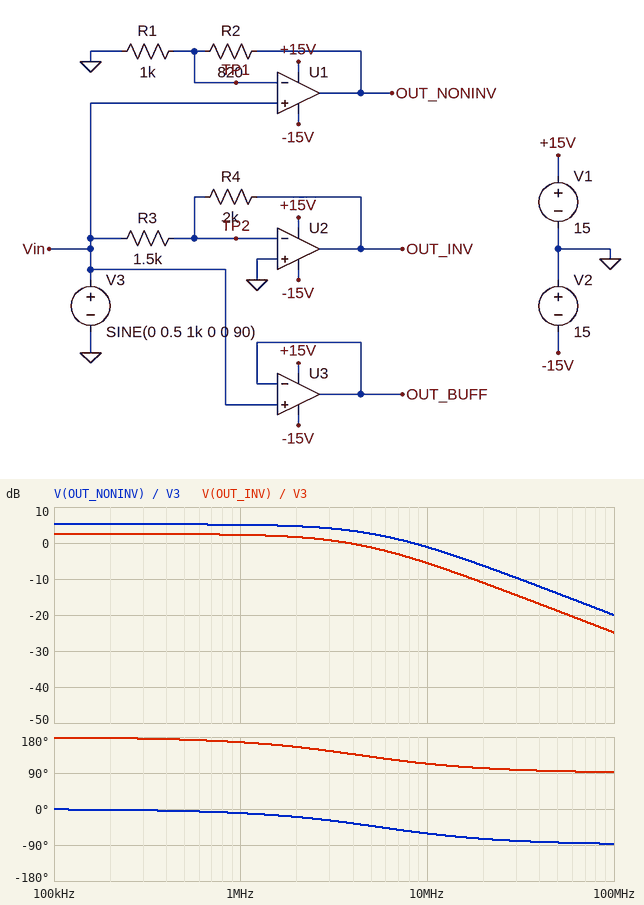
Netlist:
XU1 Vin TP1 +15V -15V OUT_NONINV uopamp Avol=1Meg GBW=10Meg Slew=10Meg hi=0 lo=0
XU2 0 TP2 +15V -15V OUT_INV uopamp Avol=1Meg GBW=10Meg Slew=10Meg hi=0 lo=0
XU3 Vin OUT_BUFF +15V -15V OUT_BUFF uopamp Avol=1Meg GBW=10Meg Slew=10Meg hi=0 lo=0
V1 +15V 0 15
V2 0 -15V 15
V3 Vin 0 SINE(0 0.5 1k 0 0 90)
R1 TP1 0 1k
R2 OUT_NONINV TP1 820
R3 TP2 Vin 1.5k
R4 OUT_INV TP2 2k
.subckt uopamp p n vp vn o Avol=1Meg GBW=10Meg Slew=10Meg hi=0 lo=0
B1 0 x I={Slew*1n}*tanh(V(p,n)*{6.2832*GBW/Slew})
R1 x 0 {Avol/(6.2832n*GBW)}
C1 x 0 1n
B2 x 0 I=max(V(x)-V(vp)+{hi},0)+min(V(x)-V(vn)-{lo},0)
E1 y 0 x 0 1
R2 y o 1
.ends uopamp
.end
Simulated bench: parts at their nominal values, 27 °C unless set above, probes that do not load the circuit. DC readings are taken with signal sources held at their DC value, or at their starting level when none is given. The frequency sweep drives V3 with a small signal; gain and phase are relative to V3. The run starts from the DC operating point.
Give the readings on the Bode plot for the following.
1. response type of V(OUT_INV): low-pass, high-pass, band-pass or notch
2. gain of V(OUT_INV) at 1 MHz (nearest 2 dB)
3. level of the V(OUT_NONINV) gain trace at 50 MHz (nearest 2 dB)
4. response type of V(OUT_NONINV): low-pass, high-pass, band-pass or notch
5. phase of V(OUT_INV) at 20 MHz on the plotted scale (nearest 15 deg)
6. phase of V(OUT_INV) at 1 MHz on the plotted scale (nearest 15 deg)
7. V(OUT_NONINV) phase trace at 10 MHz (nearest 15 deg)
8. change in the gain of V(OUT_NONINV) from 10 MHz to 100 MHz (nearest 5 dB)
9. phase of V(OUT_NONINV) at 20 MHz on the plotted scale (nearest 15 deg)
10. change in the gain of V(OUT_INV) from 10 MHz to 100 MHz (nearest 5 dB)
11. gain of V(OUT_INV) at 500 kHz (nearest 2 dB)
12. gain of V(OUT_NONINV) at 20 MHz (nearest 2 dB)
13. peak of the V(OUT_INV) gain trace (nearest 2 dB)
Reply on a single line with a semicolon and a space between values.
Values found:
low-pass; 2 dB; -14 dB; low-pass; 105 deg; 165 deg; -60 deg; -20 dB; -75 deg; -20 dB; 2 dB; -6 dB; 2 dB
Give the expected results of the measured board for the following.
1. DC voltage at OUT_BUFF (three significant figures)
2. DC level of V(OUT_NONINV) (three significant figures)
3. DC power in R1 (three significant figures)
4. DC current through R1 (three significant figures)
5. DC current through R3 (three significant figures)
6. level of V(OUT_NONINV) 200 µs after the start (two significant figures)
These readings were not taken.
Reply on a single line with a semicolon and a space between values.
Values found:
500 mV; 910 mV; 250 µW; 500 µA; 333 µA; 280 mV
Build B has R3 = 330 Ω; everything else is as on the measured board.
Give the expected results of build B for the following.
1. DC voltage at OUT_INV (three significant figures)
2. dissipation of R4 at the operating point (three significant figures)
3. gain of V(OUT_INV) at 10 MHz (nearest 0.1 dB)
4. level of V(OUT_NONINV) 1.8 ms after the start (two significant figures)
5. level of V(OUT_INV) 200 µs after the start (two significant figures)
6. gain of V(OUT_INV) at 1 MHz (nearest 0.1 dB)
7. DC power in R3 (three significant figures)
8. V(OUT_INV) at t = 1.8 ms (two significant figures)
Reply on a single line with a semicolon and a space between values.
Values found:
-3.03 V; 4.59 mW; -1.4 dB; 280 mV; -940 mV; 13.9 dB; 758 µW; -930 mV
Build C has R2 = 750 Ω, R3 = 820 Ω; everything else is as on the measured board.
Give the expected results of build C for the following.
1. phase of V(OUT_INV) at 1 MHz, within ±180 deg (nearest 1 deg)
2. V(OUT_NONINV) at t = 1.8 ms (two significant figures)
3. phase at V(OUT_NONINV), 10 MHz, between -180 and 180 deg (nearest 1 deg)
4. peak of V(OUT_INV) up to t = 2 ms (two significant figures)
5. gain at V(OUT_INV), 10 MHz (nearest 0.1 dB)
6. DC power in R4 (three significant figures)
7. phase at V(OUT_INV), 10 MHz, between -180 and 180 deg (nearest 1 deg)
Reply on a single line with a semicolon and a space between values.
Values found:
161 deg; 270 mV; -60 deg; 1.2 V; -3.3 dB; 744 µW; 106 deg
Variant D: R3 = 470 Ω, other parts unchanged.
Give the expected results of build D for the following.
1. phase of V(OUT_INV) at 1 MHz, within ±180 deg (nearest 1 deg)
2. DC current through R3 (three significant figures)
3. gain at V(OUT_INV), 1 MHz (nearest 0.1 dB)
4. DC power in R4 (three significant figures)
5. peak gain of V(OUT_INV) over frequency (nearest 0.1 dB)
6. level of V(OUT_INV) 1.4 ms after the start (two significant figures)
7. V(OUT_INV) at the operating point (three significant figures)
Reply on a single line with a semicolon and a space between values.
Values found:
152 deg; 1.06 mA; 11.5 dB; 2.26 mW; 12.6 dB; 1.7 V; -2.13 V
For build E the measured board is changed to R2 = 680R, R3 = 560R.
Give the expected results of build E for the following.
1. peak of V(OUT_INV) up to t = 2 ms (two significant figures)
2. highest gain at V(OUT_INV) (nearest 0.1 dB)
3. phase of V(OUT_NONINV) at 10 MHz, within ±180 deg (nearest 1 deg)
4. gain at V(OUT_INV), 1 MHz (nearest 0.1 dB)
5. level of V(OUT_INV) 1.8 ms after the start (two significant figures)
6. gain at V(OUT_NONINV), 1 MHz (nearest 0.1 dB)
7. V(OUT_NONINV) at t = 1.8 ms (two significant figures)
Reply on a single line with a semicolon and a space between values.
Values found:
1.8 V; 11.1 dB; -59 deg; 10.2 dB; -550 mV; 4.4 dB; 260 mV
